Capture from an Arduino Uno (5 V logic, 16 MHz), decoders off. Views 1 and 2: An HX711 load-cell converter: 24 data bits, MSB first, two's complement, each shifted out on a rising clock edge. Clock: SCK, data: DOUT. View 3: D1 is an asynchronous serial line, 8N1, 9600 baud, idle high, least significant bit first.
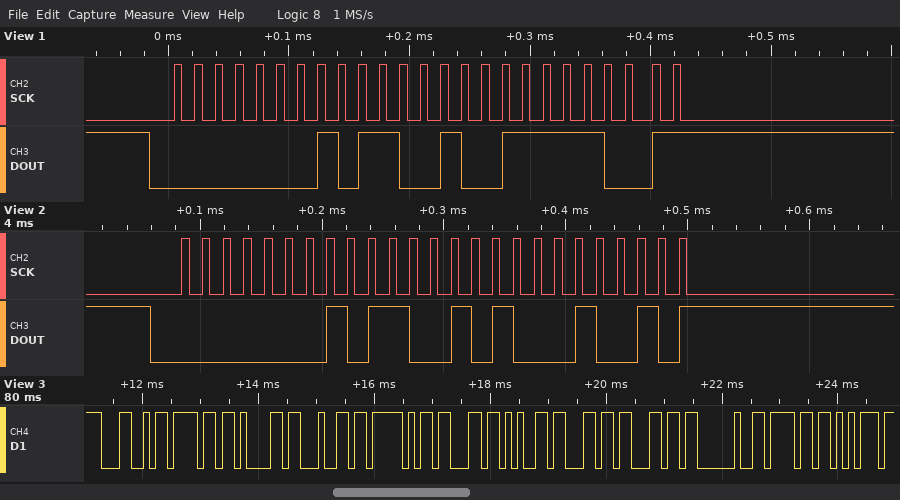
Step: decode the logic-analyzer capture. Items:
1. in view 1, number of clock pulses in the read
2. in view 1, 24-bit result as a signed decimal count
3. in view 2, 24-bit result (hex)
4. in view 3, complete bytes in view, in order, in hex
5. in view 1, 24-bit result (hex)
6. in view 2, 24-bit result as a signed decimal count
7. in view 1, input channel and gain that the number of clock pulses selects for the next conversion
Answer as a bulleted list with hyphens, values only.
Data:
- 25
- 91385
- 0x016512
- 4C 6F 61 64 5F 63 65 6C 6C 20 6F 75
- 0x0164F9
- 91410
- channel A, gain 128
